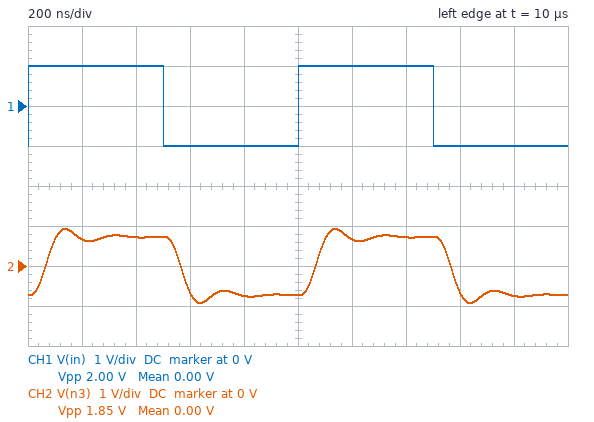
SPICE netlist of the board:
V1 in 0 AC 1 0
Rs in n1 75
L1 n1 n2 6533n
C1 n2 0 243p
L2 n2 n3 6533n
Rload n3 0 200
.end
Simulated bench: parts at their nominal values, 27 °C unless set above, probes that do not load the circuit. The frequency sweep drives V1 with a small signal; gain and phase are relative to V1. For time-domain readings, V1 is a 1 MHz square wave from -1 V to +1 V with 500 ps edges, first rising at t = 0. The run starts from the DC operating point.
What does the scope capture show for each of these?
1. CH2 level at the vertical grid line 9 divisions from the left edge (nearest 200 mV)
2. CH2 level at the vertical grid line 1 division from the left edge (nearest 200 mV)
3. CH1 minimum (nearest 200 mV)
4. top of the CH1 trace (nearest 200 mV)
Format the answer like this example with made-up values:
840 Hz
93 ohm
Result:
-800 mV
600 mV
-1.0 V
1.0 V
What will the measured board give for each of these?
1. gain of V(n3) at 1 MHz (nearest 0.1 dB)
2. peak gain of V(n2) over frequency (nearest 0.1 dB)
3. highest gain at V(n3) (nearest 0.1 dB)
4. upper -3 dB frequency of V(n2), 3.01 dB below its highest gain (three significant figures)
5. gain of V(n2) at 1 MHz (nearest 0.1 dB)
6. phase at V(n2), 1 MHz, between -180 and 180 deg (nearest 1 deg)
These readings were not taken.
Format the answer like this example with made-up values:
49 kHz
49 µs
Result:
-2.8 dB
1.0 dB
-1.9 dB
6.32 MHz
-2.7 dB
-10 deg
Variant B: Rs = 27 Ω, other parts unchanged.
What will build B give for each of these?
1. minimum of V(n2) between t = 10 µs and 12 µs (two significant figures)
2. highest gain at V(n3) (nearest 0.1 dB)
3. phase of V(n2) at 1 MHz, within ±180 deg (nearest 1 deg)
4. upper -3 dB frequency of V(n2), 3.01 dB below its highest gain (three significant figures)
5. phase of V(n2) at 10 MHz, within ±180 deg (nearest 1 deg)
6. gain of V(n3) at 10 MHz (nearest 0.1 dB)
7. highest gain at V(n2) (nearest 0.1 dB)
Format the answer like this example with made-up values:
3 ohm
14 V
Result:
-1.4 V
0.9 dB
-11 deg
6.00 MHz
-170 deg
-20.2 dB
3.9 dB
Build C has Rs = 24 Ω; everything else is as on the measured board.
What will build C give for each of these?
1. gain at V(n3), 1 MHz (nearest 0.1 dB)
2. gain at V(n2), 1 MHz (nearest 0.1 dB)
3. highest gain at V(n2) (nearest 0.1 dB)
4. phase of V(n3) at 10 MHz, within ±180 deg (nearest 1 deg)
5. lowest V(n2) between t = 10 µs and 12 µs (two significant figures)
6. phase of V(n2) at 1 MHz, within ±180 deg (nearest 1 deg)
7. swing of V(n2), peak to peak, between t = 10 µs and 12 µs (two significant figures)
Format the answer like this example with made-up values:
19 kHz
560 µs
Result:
-1.1 dB
-0.9 dB
4.1 dB
125 deg
-1.5 V
-11 deg
2.9 V
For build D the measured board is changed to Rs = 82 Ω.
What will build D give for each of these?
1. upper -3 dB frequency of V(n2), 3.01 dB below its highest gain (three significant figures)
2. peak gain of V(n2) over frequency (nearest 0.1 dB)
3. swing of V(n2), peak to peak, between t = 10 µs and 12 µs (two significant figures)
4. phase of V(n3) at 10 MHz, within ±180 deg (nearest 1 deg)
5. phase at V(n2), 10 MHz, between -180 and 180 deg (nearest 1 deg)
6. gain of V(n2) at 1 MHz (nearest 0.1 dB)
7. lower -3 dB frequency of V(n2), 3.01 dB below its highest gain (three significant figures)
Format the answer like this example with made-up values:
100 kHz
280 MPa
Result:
6.36 MHz
0.6 dB
2.2 V
135 deg
-161 deg
-2.9 dB
2.10 MHz
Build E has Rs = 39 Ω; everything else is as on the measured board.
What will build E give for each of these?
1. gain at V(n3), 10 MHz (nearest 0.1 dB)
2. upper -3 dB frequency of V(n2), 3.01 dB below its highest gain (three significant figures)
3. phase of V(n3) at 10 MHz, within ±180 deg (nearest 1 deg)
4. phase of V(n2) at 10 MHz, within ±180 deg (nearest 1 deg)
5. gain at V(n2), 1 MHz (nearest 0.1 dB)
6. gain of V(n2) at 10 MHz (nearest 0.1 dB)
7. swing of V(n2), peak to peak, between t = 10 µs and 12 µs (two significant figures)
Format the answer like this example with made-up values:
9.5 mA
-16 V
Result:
-20.3 dB
6.09 MHz
128 deg
-168 deg
-1.5 dB
-13.1 dB
2.7 V
